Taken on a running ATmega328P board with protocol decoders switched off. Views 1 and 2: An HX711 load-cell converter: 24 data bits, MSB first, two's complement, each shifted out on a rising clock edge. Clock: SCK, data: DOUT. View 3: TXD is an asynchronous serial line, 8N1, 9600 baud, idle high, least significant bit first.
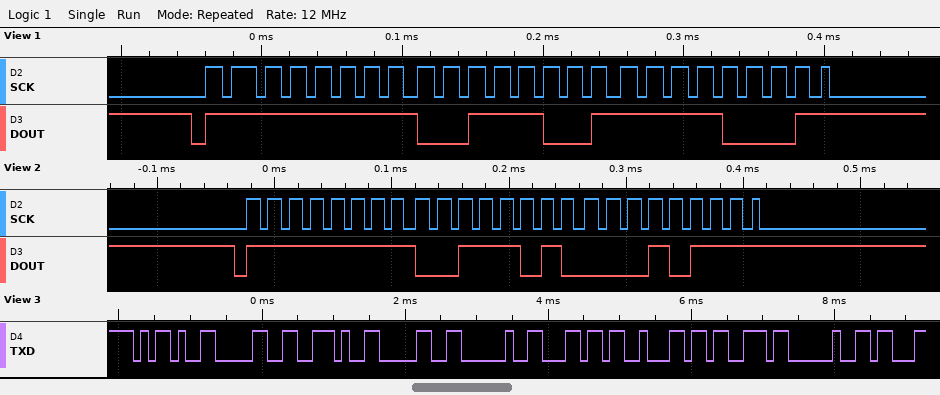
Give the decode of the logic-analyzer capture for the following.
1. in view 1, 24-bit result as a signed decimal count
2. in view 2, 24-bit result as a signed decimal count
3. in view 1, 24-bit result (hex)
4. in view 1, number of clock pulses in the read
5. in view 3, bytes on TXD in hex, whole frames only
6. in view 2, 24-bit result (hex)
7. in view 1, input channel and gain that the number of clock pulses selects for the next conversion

-50703
-50665
0xFF39F1
25
2D 30 2E 30 20 6C 62 73 20
0xFF3A17
channel A, gain 128
